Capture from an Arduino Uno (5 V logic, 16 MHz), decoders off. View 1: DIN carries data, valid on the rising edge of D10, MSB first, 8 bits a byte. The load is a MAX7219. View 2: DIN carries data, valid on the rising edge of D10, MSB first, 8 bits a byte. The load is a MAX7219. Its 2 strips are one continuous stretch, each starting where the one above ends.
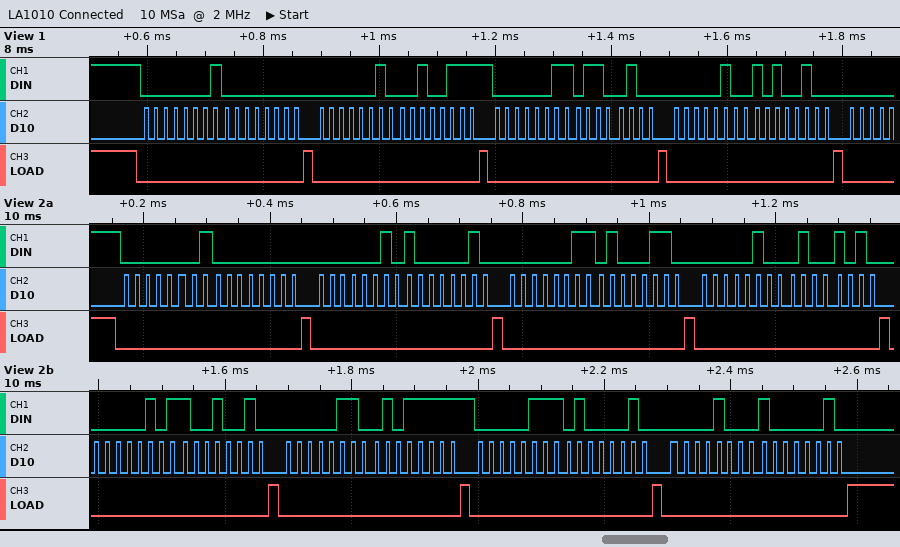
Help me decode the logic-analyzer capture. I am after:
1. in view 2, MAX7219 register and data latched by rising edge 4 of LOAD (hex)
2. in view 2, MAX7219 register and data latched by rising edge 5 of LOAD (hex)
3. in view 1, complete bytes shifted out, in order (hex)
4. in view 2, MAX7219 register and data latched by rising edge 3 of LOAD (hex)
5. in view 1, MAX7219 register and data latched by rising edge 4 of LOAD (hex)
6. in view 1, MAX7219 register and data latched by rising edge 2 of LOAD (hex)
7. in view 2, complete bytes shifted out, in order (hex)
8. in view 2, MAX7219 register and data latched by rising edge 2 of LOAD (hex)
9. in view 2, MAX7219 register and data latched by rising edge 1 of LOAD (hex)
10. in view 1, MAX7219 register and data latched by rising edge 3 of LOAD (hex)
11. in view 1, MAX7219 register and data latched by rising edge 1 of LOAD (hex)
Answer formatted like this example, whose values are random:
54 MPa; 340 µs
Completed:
register 0x4, data 0x4A; register 0x5, data 0x92; 01 00 02 27 03 64 04 A4; register 0x3, data 0x46; register 0x4, data 0xA4; register 0x2, data 0x27; 01 00 02 82 03 46 04 4A 05 92 06 5F 07 42 08 82; register 0x2, data 0x82; register 0x1, data 0x00; register 0x3, data 0x64; register 0x1, data 0x00
